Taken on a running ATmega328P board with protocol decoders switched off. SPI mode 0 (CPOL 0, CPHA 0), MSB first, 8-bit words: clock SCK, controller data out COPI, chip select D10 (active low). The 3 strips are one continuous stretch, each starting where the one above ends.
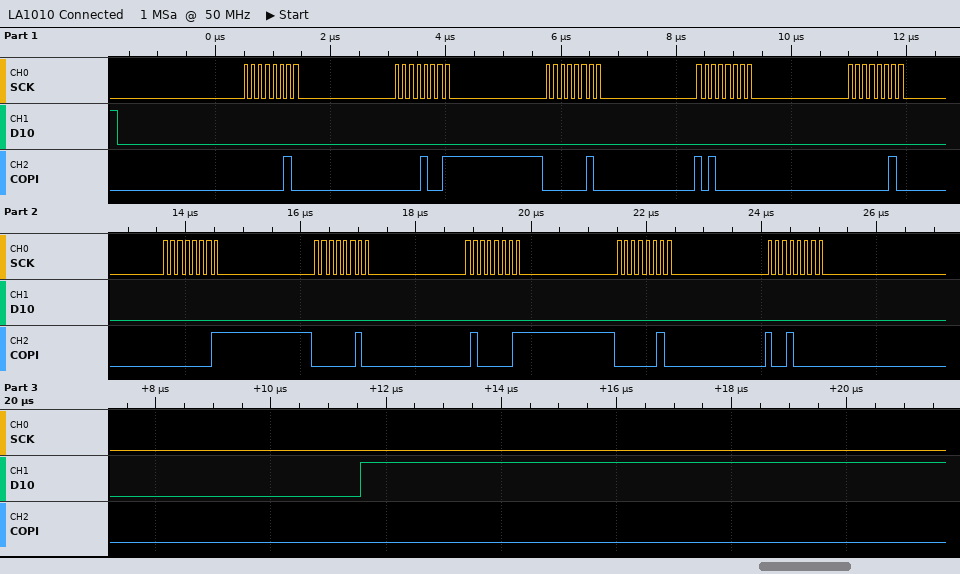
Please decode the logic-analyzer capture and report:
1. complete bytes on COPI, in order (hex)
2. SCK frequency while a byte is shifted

02 09 02 A0 02 01 02 41 02 90
8 MHz
